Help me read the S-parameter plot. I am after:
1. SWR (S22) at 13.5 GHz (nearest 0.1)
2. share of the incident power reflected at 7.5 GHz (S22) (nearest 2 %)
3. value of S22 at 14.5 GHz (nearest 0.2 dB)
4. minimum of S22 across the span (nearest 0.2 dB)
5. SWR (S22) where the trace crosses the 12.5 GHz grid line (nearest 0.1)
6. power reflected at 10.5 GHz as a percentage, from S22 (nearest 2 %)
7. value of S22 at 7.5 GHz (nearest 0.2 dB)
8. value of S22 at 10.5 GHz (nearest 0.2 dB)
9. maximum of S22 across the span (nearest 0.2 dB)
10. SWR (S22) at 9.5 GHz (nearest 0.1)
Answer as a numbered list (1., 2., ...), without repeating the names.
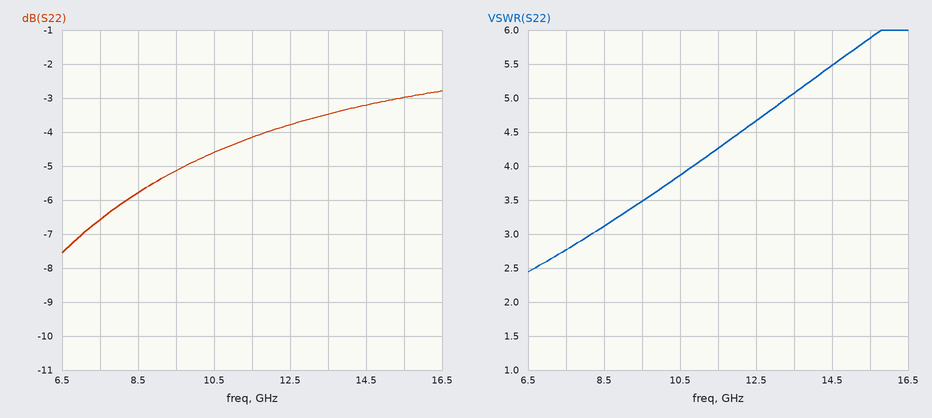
1. 5.1
2. 22 %
3. -3.2 dB
4. -7.6 dB
5. 4.7
6. 34 %
7. -6.6 dB
8. -4.6 dB
9. -2.8 dB
10. 3.5
